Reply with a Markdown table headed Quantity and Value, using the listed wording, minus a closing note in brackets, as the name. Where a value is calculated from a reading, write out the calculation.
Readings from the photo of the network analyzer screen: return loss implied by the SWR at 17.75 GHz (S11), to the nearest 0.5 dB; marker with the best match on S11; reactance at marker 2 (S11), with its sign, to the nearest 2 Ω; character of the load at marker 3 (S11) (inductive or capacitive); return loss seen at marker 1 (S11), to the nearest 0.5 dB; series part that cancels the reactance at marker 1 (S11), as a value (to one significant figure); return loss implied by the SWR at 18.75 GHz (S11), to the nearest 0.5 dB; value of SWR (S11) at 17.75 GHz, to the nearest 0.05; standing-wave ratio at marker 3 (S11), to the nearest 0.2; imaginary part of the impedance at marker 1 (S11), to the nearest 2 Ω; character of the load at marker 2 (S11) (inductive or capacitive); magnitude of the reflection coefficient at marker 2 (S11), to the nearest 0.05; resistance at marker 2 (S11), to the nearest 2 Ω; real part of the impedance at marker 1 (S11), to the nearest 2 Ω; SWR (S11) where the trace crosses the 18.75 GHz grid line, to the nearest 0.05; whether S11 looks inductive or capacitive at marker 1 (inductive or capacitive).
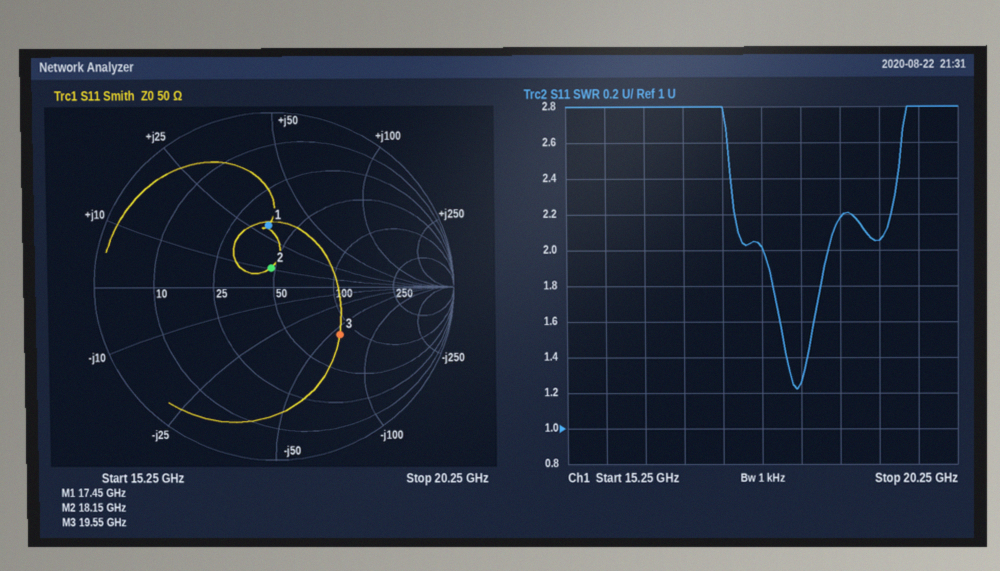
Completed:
| Quantity | Value |
|---|---|
| return loss implied by the SWR at 17.75 GHz (S11), to the nearest 0.5 dB | −20 log10((2 − 1)/(2 + 1)) ≈ 9.5 dB |
| marker with the best match on S11 | marker 2 |
| reactance at marker 2 (S11), with its sign, to the nearest 2 Ω | +10 Ω |
| character of the load at marker 3 (S11) | capacitive |
| return loss seen at marker 1 (S11), to the nearest 0.5 dB | 9.0 dB |
| series part that cancels the reactance at marker 1 (S11), as a value | C = 1/(2π × 17.45 GHz × 30 Ω) ≈ 304 fF, so 300 fF to one significant figure |
| return loss implied by the SWR at 18.75 GHz (S11), to the nearest 0.5 dB | −20 log10((2.2 − 1)/(2.2 + 1)) ≈ 8.5 dB |
| value of SWR (S11) at 17.75 GHz, to the nearest 0.05 | 2.00 |
| standing-wave ratio at marker 3 (S11), to the nearest 0.2 | 2.6 |
| imaginary part of the impedance at marker 1 (S11), to the nearest 2 Ω | +30 Ω |
| character of the load at marker 2 (S11) | inductive |
| magnitude of the reflection coefficient at marker 2 (S11), to the nearest 0.05 | 0.10 |
| resistance at marker 2 (S11), to the nearest 2 Ω | 48 Ω |
| real part of the impedance at marker 1 (S11), to the nearest 2 Ω | 38 Ω |
| SWR (S11) where the trace crosses the 18.75 GHz grid line, to the nearest 0.05 | 2.20 |
| whether S11 looks inductive or capacitive at marker 1 | inductive |
